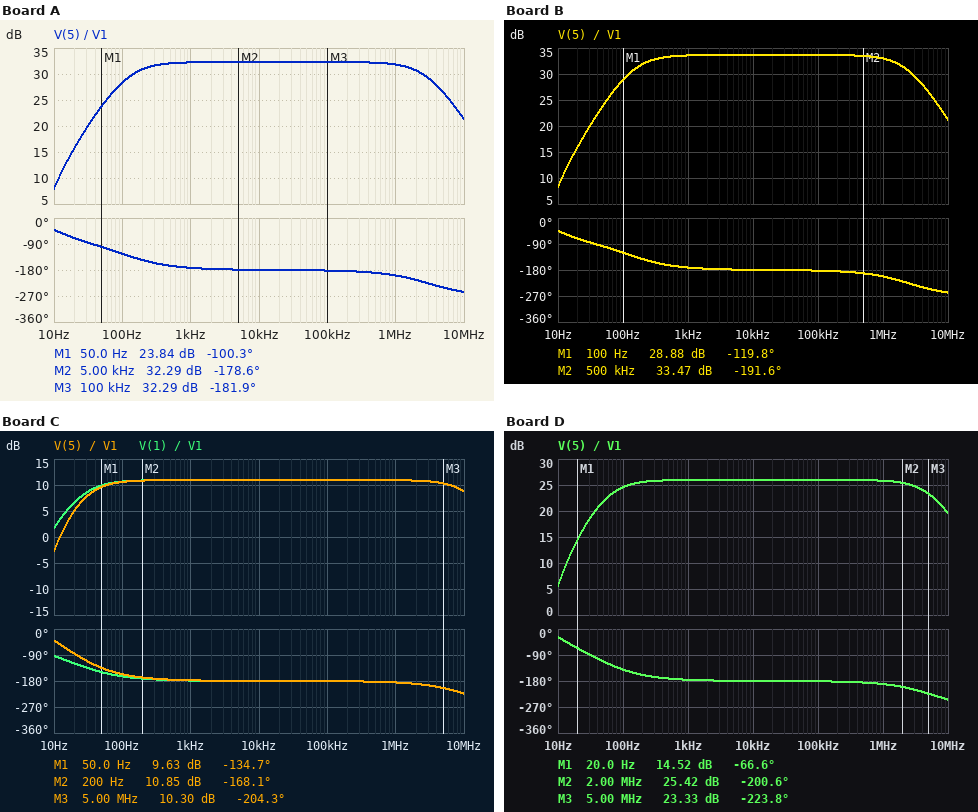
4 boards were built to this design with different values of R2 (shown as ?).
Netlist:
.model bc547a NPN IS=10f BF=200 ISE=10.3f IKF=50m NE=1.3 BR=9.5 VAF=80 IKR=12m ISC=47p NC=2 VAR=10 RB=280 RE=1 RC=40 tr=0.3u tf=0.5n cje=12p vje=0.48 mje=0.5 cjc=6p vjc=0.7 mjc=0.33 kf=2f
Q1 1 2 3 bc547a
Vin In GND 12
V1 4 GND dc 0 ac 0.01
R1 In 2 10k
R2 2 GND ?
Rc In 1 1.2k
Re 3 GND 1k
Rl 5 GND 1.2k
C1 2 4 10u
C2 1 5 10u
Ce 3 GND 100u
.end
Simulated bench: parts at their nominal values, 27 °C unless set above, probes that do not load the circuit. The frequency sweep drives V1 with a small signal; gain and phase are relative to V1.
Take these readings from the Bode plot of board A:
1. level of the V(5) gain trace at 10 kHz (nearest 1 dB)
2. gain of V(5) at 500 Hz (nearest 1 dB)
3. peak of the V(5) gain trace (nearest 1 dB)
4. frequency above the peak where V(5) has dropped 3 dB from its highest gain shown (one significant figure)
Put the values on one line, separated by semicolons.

32 dB; 32 dB; 32 dB; 3 MHz
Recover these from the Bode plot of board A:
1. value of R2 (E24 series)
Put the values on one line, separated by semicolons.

3.6 kΩ
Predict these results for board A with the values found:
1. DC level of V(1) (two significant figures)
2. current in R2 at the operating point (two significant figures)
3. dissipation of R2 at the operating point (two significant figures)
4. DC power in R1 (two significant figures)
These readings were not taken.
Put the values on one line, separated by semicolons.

9.1 V; 870 µA; 2.7 mW; 7.9 mW
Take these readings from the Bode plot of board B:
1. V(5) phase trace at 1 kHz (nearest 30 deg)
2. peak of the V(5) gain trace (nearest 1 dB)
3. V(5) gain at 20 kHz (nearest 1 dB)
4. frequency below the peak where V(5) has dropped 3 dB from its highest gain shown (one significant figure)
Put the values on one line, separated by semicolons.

-180 deg; 34 dB; 34 dB; 100 Hz
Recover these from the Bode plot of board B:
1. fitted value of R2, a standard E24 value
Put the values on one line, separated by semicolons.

4.7 kΩ
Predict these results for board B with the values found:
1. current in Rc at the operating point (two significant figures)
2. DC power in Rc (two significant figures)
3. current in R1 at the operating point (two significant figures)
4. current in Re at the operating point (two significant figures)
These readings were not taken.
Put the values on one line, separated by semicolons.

3.0 mA; 11 mW; 820 µA; 3.1 mA
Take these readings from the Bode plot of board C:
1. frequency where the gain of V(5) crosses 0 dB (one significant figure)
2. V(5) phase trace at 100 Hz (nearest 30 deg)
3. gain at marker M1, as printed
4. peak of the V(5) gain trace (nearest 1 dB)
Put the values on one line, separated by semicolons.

10 Hz; -150 deg; 9.63 dB; 11 dB
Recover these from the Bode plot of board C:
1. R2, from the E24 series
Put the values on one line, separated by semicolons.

680 Ω
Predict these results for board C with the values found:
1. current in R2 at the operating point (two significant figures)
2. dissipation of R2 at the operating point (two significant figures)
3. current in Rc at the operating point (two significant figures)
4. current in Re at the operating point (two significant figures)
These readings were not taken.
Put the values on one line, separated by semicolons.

1.1 mA; 860 µW; 160 µA; 160 µA
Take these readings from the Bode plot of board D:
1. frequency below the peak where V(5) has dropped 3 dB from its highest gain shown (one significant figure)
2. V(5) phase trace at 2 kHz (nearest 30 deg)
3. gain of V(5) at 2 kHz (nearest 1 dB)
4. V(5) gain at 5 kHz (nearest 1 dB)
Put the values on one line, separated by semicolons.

60 Hz; -180 deg; 26 dB; 26 dB
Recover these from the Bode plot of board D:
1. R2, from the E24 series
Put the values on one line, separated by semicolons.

1.6 kΩ
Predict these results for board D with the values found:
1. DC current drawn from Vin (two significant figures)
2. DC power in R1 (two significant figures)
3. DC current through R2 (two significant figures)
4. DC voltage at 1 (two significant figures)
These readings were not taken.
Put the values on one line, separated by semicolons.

2.0 mA; 11 mW; 1.0 mA; 11 V
